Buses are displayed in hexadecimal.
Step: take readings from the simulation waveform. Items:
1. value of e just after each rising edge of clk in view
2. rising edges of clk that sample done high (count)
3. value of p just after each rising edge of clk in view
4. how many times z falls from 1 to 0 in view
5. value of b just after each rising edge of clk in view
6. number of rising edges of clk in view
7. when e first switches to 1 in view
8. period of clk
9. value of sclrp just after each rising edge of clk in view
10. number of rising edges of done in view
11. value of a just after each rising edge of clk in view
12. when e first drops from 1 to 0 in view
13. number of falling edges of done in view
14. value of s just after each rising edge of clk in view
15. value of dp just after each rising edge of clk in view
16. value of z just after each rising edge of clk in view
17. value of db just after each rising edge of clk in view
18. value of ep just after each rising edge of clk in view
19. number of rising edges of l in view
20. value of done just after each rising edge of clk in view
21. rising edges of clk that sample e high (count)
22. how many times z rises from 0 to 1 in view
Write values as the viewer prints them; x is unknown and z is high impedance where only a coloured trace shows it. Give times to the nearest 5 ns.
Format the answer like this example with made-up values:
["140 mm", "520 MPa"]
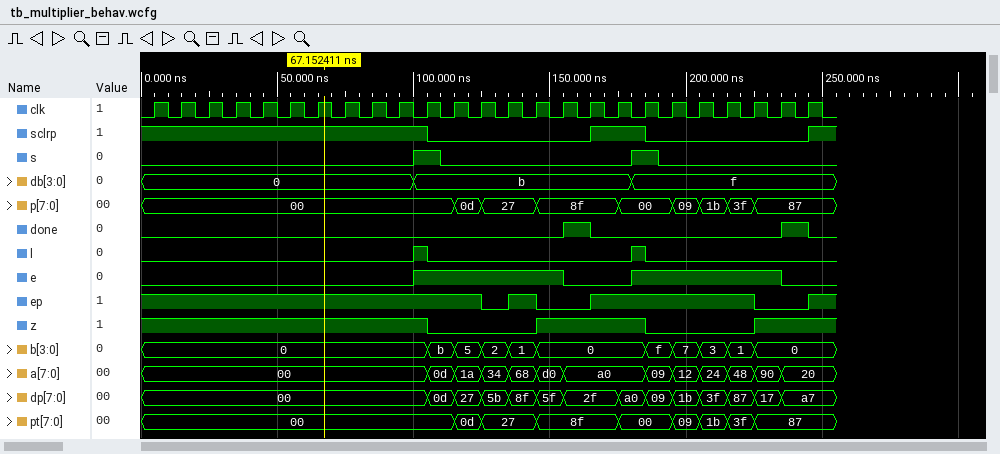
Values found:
["0 0 0 0 0 0 0 0 0 0 1 1 1 1 1 0 0 0 1 1 1 1 1 0 0", "2", "00, 00, 00, 00, 00, 00, 00, 00, 00, 00, 00, 0d, 27, 27, 8f, 8f, 8f, 00, 00, 09, 1b, 3f, 87, 87, 87", "2", "0, 0, 0, 0, 0, 0, 0, 0, 0, 0, b, 5, 2, 1, 0, 0, 0, 0, f, 7, 3, 1, 0, 0, 0", "25", "100 ns", "10 ns", "1 1 1 1 1 1 1 1 1 1 0 0 0 0 0 0 1 1 0 0 0 0 0 0 1", "2", "00, 00, 00, 00, 00, 00, 00, 00, 00, 00, 0d, 1a, 34, 68, d0, a0, a0, a0, 09, 12, 24, 48, 90, 20, 20", "155 ns", "2", "0 0 0 0 0 0 0 0 0 0 1 0 0 0 0 0 0 0 1 0 0 0 0 0 0", "00, 00, 00, 00, 00, 00, 00, 00, 00, 00, 0d, 27, 5b, 8f, 5f, 2f, 2f, a0, 09, 1b, 3f, 87, 17, a7, a7", "1 1 1 1 1 1 1 1 1 1 0 0 0 0 1 1 1 1 0 0 0 0 1 1 1", "0, 0, 0, 0, 0, 0, 0, 0, 0, 0, b, b, b, b, b, b, b, b, f, f, f, f, f, f, f", "1 1 1 1 1 1 1 1 1 1 1 1 0 1 0 0 1 1 1 1 1 1 0 0 1", "2", "0 0 0 0 0 0 0 0 0 0 0 0 0 0 0 1 0 0 0 0 0 0 0 1 0", "12", "2"]
